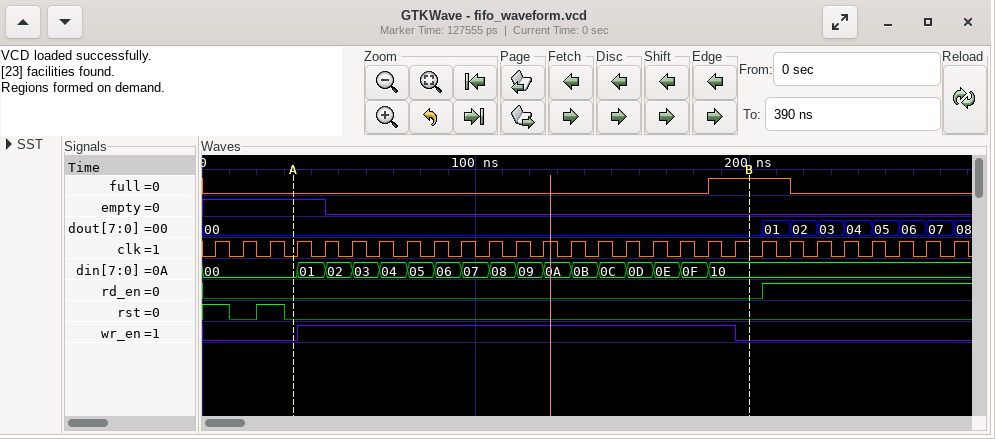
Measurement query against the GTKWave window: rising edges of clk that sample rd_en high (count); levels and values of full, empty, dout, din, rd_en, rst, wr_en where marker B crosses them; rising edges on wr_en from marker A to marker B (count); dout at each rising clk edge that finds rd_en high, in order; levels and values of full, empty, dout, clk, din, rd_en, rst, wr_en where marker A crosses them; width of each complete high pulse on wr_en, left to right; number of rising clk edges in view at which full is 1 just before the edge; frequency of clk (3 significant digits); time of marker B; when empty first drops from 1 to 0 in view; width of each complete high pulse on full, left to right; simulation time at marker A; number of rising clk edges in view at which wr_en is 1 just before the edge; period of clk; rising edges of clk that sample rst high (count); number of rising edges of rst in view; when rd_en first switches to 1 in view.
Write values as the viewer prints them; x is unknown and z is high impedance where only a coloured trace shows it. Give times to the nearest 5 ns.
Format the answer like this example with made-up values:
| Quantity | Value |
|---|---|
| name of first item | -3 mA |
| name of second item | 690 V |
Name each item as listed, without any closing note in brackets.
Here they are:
| Quantity | Value |
|---|---|
| rising edges of clk that sample rd_en high | 7 |
| levels and values of full, empty, dout, din, rd_en, rst, wr_en where marker B crosses them | full=1, empty=0, dout=00, din=10, rd_en=0, rst=0, wr_en=0 |
| rising edges on wr_en from marker A to marker B | 1 |
| dout at each rising clk edge that finds rd_en high, in order | 01, 02, 03, 04, 05, 06, 07 |
| levels and values of full, empty, dout, clk, din, rd_en, rst, wr_en where marker A crosses them | full=0, empty=1, dout=00, clk=0, din=00, rd_en=0, rst=0, wr_en=0 |
| width of each complete high pulse on wr_en, left to right | 160 ns |
| number of rising clk edges in view at which full is 1 just before the edge | 3 |
| frequency of clk | 100 MHz |
| time of marker B | 200 ns |
| when empty first drops from 1 to 0 in view | 45 ns |
| width of each complete high pulse on full, left to right | 30 ns |
| simulation time at marker A | 35 ns |
| number of rising clk edges in view at which wr_en is 1 just before the edge | 16 |
| period of clk | 10 ns |
| rising edges of clk that sample rst high | 2 |
| number of rising edges of rst in view | 1 |
| when rd_en first switches to 1 in view | 205 ns |
